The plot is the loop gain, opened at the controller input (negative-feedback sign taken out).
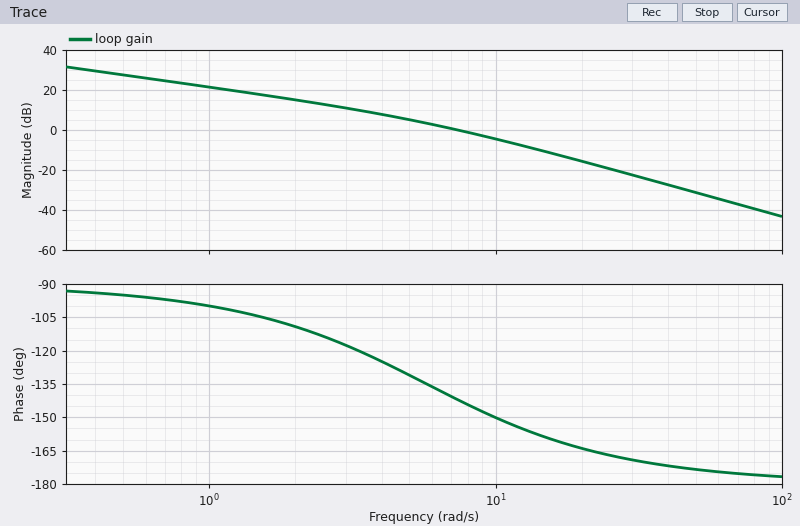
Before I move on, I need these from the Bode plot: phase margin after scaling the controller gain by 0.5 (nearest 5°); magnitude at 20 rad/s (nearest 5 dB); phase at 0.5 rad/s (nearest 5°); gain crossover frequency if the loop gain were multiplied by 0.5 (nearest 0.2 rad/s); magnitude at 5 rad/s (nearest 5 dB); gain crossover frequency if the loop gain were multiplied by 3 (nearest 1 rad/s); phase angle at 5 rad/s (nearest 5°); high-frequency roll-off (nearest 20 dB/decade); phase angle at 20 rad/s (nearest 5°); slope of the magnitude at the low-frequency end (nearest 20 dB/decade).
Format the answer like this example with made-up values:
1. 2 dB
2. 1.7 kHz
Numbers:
1. 50°
2. -15 dB
3. -95°
4. 4.6 rad/s
5. 5 dB
6. 14 rad/s
7. -130°
8. -40 dB/decade
9. -165°
10. -20 dB/decade
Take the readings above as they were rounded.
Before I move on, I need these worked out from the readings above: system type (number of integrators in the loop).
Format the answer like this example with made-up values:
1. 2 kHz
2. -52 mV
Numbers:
1. 1
